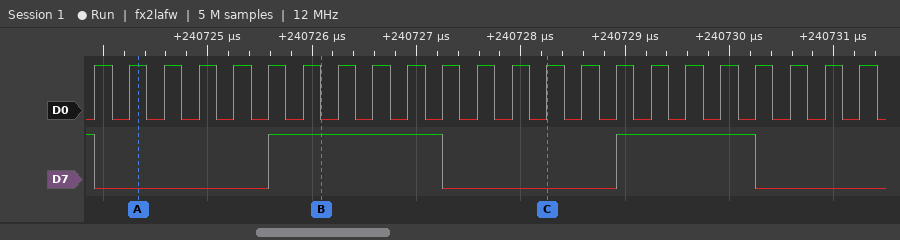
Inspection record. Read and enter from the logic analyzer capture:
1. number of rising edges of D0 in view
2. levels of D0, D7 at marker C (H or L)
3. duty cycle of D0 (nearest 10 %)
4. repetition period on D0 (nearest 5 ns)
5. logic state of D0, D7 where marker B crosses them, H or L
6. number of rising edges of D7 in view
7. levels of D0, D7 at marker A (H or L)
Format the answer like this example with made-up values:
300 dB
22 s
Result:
23
D0=H, D7=L
50 %
335 ns
D0=L, D7=H
2
D0=H, D7=L
